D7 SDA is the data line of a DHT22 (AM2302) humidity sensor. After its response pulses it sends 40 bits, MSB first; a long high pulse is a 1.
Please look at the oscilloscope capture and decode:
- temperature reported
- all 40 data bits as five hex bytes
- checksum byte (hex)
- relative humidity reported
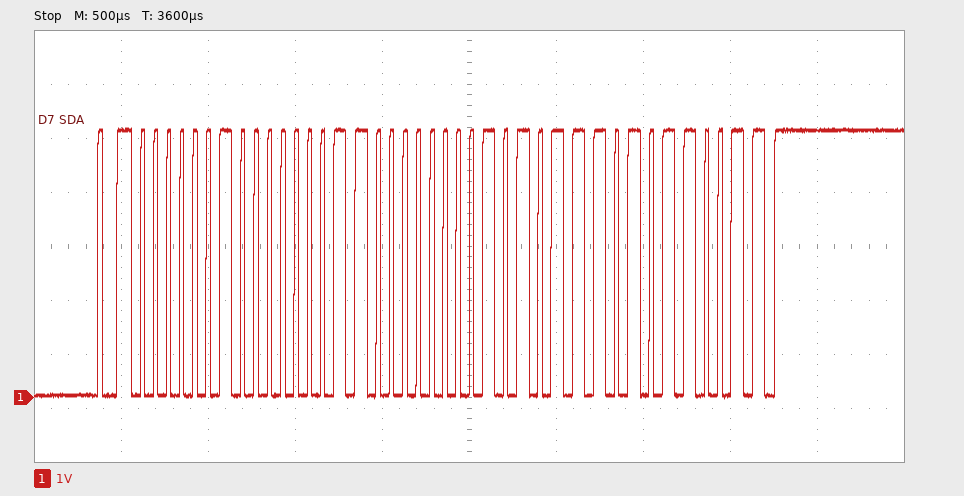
17.4 °C
02 03 00 AE B3
0xB3
51.5 %
